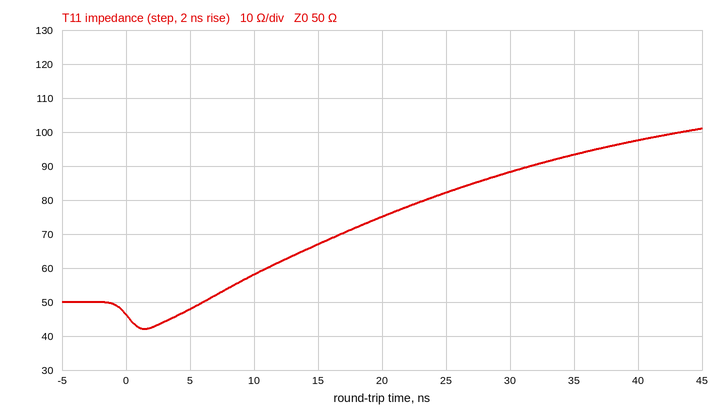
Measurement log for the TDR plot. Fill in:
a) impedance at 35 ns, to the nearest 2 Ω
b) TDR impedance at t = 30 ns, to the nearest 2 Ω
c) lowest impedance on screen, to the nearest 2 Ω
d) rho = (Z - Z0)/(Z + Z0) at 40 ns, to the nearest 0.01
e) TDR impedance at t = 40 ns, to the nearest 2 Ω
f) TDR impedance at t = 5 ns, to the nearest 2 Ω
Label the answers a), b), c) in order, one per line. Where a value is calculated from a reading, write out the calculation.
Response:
a) 94 Ω
b) 88 Ω
c) 42 Ω
d) (98 − 50)/(98 + 50) ≈ +0.32
e) 98 Ω
f) 48 Ω
